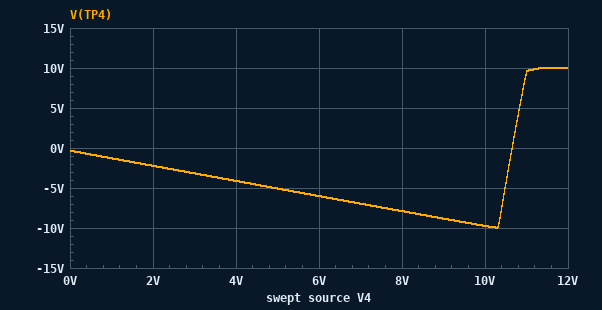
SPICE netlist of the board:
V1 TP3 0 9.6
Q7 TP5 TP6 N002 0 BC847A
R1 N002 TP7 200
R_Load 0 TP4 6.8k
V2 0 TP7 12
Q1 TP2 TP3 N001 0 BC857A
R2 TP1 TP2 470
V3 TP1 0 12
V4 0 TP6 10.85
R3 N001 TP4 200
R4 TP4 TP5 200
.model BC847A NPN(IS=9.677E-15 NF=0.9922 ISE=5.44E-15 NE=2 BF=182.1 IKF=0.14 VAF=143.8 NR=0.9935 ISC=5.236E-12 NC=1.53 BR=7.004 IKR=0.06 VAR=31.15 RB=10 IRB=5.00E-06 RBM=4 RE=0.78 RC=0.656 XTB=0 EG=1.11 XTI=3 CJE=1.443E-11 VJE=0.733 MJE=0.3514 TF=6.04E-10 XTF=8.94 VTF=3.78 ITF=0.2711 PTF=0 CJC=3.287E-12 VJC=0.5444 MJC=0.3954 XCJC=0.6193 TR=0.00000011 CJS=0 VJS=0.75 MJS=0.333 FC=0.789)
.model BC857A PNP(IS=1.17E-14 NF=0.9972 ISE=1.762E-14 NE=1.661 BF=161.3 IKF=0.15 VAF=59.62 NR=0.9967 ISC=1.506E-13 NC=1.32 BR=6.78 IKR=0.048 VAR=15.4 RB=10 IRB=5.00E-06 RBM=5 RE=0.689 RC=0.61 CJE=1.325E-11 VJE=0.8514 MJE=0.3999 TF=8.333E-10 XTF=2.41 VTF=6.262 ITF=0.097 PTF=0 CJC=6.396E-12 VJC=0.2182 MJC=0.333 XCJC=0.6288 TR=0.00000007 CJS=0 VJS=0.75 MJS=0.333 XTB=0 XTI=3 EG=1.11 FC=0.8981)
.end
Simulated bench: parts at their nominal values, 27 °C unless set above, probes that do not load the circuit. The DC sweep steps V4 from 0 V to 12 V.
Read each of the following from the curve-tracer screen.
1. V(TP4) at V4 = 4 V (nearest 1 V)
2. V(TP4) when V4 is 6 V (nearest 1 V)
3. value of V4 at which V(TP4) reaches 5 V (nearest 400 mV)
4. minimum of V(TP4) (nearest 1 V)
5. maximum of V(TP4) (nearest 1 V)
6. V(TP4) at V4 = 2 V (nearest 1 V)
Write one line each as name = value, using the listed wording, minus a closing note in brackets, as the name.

V(TP4) at V4 = 4 V = -4 V
V(TP4) when V4 is 6 V = -6 V
value of V4 at which V(TP4) reaches 5 V = 10.8 V
minimum of V(TP4) = -10 V
maximum of V(TP4) = 10 V
V(TP4) at V4 = 2 V = -2 V
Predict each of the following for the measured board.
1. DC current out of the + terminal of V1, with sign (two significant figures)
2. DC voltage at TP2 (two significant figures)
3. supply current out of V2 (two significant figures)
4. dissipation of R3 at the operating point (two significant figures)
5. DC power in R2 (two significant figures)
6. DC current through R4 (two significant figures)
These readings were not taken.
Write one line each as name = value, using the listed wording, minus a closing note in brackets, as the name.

DC current out of the + terminal of V1, with sign = -470 µA
DC voltage at TP2 = 10 V
supply current out of V2 = 2.4 mA
dissipation of R3 at the operating point = 2.0 mW
DC power in R2 = 6.3 mW
DC current through R4 = 2.4 mA
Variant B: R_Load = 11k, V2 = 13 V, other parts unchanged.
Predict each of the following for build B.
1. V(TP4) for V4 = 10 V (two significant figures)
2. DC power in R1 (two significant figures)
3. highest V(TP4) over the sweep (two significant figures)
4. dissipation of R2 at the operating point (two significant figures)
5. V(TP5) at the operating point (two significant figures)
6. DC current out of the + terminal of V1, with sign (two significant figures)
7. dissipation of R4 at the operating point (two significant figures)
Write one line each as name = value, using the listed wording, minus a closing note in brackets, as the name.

V(TP4) for V4 = 10 V = -9.9 V
DC power in R1 = 9.8 mW
highest V(TP4) over the sweep = 9.8 V
dissipation of R2 at the operating point = 6.4 mW
V(TP5) at the operating point = -12 V
DC current out of the + terminal of V1, with sign = -270 µA
dissipation of R4 at the operating point = 3.9 mW
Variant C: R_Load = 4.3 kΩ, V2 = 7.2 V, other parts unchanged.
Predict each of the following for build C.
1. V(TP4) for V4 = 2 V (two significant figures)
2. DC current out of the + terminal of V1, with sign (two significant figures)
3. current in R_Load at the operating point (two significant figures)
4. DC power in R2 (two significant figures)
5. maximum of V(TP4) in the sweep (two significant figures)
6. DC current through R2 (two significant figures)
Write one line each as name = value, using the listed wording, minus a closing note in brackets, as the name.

V(TP4) for V4 = 2 V = -2.1 V
DC current out of the + terminal of V1, with sign = -1.3 mA
current in R_Load at the operating point = 2.3 mA
DC power in R2 = 6.1 mW
maximum of V(TP4) in the sweep = 9.8 V
DC current through R2 = 3.6 mA
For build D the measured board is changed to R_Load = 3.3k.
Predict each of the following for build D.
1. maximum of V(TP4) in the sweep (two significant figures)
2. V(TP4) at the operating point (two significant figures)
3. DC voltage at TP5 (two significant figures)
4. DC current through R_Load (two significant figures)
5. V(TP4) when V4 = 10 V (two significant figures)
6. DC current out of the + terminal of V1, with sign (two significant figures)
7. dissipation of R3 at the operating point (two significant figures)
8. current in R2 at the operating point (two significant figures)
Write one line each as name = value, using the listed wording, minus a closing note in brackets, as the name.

maximum of V(TP4) in the sweep = 9.7 V
V(TP4) at the operating point = 2.9 V
DC voltage at TP5 = 2.4 V
DC current through R_Load = 880 µA
V(TP4) when V4 = 10 V = -9.4 V
DC current out of the + terminal of V1, with sign = -420 µA
dissipation of R3 at the operating point = 2.1 mW
current in R2 at the operating point = 3.7 mA
